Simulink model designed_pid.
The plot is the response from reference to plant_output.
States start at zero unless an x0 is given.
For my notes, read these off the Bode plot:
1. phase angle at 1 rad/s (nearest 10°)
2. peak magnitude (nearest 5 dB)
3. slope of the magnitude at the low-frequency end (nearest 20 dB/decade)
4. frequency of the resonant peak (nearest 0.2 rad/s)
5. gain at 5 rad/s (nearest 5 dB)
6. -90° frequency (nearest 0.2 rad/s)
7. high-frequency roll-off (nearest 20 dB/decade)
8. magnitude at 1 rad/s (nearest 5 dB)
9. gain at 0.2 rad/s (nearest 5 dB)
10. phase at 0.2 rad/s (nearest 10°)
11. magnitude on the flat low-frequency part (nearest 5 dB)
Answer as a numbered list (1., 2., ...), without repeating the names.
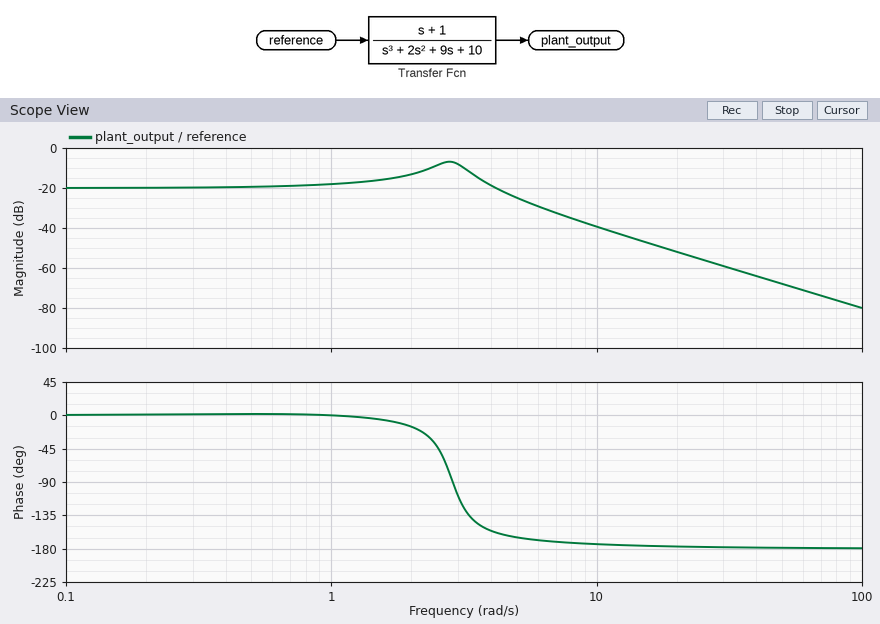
1. 0°
2. -5 dB
3. 0 dB/decade
4. 2.8 rad/s
5. -25 dB
6. 2.8 rad/s
7. -40 dB/decade
8. -20 dB
9. -20 dB
10. 0°
11. -20 dB
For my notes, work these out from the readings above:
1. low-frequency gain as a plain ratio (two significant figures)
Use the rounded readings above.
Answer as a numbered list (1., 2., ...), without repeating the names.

1. 0.10
